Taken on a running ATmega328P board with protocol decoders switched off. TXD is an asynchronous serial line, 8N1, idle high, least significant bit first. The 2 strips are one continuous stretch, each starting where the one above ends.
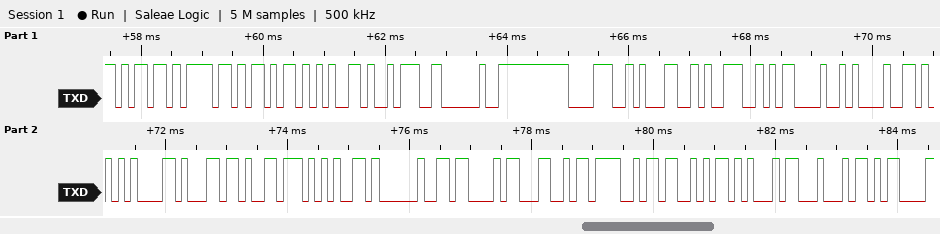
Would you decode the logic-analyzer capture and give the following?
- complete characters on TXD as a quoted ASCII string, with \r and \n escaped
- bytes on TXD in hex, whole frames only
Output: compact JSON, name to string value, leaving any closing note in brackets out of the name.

{"complete characters on TXD as a quoted ASCII string, with \\r and \\n escaped": "\"moke: 819\\r\\nValve CLOSED\\r\"", "bytes on TXD in hex, whole frames only": "6D 6F 6B 65 3A 20 38 31 39 0D 0A 56 61 6C 76 65 20 43 4C 4F 53 45 44 0D"}
